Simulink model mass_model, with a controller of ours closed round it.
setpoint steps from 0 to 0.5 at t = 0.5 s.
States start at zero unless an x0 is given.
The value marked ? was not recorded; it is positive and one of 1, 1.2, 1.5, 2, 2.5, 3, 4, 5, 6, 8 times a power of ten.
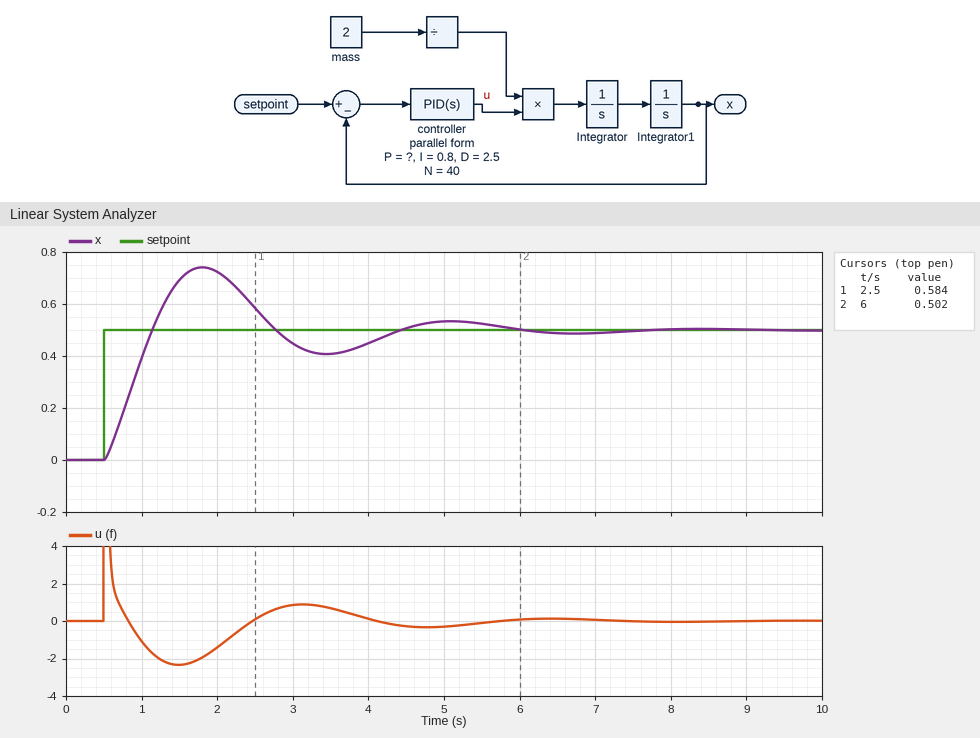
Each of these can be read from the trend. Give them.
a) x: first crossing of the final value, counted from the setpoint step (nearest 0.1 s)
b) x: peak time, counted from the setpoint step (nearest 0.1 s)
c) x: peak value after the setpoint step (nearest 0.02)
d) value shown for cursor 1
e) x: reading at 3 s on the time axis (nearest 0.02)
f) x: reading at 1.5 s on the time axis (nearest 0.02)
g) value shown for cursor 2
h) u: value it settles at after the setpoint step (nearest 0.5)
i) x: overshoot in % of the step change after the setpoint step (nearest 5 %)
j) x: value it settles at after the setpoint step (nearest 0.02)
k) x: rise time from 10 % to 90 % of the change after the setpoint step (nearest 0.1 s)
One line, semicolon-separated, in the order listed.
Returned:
0.6 s; 1.3 s; 0.74; 0.584; 0.44; 0.70; 0.502; 0.0; 50 %; 0.50; 0.5 s
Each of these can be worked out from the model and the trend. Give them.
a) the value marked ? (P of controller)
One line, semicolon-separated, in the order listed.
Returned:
8
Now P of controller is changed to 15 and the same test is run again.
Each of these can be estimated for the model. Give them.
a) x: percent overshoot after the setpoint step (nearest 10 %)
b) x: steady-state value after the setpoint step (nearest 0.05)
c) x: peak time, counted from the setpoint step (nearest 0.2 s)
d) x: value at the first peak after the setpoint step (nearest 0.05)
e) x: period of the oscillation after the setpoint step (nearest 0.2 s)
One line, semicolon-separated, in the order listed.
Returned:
60 %; 0.50; 1.0 s; 0.80; 2.4 s
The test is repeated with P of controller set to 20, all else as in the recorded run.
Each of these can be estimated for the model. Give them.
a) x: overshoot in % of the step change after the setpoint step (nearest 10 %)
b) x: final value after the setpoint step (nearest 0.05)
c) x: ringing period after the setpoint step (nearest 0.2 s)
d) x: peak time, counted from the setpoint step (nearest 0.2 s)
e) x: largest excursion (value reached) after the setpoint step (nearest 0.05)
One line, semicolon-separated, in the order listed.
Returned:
60 %; 0.50; 2.0 s; 0.8 s; 0.80
